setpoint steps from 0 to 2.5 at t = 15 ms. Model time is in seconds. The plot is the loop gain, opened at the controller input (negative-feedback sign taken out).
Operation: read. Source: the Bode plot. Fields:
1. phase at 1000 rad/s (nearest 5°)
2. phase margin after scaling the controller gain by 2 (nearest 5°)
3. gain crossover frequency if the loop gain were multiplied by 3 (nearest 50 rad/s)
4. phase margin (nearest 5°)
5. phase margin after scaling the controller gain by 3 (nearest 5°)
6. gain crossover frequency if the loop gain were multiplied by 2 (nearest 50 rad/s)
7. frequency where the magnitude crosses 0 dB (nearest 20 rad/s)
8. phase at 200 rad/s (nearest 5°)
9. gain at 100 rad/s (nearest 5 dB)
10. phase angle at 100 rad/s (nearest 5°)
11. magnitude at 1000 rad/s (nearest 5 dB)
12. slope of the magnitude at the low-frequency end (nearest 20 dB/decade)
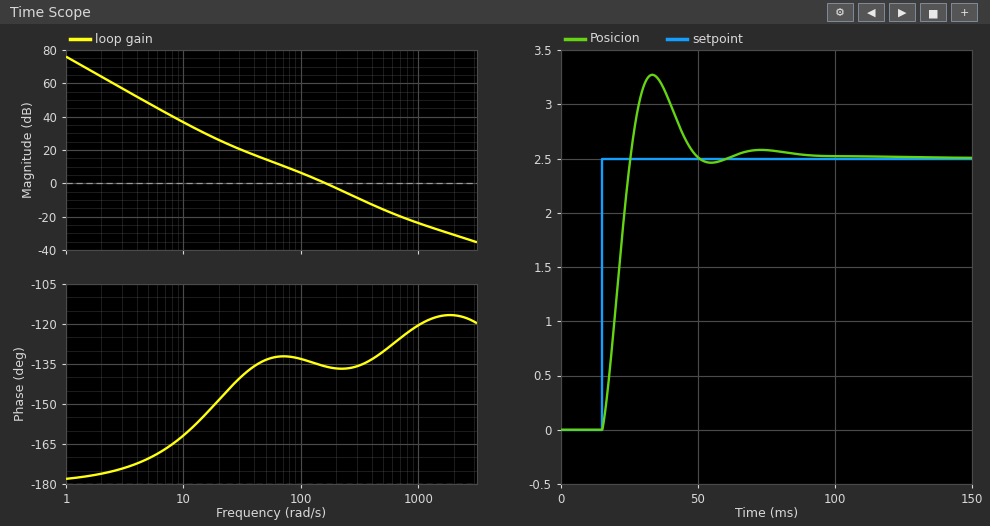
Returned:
-120°
45°
300 rad/s
45°
45°
250 rad/s
160 rad/s
-135°
5 dB
-135°
-25 dB
-40 dB/decade
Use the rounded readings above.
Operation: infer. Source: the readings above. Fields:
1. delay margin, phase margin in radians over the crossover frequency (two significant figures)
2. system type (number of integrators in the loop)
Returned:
0.0049 s
2
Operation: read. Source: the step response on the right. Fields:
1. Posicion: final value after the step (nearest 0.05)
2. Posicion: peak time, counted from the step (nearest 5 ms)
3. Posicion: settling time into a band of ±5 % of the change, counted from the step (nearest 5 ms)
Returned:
2.50
20 ms
30 ms
